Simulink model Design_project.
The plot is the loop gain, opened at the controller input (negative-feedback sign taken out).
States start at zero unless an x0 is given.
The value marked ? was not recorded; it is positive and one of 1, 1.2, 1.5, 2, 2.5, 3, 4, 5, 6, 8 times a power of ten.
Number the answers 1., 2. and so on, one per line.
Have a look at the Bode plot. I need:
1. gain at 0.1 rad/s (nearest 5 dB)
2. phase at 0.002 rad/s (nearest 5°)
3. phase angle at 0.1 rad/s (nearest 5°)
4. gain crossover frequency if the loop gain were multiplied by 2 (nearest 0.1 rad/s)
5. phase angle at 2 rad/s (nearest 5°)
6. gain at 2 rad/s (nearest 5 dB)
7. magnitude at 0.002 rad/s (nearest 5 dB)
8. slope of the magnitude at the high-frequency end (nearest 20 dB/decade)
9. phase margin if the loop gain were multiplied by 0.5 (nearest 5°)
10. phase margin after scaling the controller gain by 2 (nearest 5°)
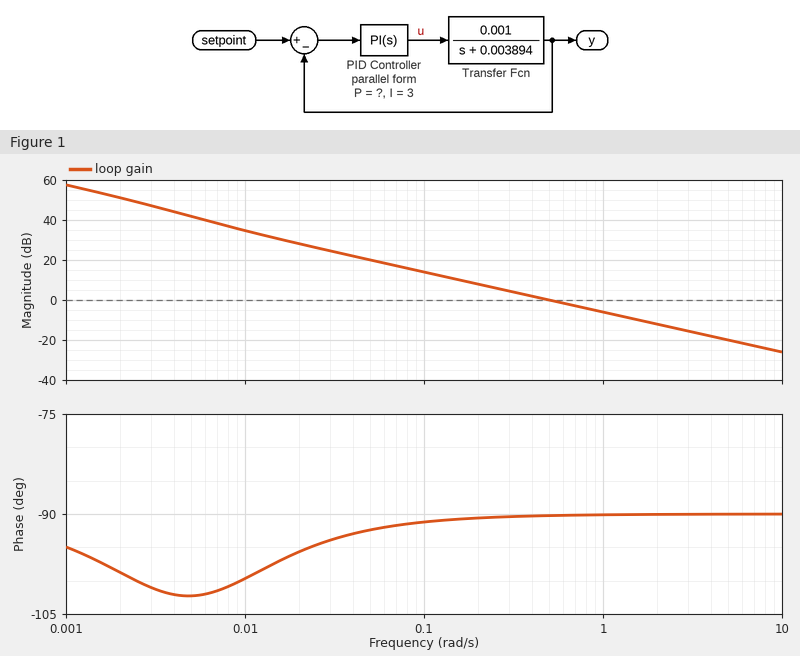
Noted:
1. 15 dB
2. -100°
3. -90°
4. 1.0 rad/s
5. -90°
6. -10 dB
7. 50 dB
8. -20 dB/decade
9. 90°
10. 90°
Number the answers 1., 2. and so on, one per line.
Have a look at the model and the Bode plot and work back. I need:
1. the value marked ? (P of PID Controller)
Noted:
1. 500
